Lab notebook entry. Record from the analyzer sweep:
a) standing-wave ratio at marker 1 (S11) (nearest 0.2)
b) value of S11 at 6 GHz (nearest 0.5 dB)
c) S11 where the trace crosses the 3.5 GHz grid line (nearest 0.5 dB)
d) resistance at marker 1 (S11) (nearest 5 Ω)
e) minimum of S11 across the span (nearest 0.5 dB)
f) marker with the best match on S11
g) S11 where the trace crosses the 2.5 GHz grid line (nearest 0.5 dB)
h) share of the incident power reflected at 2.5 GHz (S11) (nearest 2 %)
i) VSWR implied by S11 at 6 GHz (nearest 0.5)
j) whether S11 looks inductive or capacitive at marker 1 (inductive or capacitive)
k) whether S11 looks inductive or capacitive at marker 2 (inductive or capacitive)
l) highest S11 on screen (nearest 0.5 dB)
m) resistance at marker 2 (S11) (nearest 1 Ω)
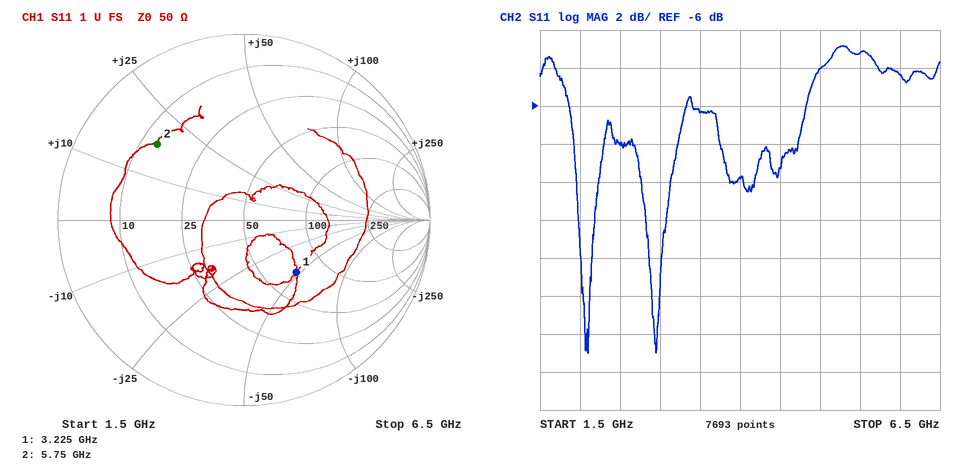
2.4
-4.5 dB
-6.5 dB
70 Ω
-19.0 dB
marker 1
-8.0 dB
16 %
4.0
capacitive
inductive
-3.0 dB
13 Ω
